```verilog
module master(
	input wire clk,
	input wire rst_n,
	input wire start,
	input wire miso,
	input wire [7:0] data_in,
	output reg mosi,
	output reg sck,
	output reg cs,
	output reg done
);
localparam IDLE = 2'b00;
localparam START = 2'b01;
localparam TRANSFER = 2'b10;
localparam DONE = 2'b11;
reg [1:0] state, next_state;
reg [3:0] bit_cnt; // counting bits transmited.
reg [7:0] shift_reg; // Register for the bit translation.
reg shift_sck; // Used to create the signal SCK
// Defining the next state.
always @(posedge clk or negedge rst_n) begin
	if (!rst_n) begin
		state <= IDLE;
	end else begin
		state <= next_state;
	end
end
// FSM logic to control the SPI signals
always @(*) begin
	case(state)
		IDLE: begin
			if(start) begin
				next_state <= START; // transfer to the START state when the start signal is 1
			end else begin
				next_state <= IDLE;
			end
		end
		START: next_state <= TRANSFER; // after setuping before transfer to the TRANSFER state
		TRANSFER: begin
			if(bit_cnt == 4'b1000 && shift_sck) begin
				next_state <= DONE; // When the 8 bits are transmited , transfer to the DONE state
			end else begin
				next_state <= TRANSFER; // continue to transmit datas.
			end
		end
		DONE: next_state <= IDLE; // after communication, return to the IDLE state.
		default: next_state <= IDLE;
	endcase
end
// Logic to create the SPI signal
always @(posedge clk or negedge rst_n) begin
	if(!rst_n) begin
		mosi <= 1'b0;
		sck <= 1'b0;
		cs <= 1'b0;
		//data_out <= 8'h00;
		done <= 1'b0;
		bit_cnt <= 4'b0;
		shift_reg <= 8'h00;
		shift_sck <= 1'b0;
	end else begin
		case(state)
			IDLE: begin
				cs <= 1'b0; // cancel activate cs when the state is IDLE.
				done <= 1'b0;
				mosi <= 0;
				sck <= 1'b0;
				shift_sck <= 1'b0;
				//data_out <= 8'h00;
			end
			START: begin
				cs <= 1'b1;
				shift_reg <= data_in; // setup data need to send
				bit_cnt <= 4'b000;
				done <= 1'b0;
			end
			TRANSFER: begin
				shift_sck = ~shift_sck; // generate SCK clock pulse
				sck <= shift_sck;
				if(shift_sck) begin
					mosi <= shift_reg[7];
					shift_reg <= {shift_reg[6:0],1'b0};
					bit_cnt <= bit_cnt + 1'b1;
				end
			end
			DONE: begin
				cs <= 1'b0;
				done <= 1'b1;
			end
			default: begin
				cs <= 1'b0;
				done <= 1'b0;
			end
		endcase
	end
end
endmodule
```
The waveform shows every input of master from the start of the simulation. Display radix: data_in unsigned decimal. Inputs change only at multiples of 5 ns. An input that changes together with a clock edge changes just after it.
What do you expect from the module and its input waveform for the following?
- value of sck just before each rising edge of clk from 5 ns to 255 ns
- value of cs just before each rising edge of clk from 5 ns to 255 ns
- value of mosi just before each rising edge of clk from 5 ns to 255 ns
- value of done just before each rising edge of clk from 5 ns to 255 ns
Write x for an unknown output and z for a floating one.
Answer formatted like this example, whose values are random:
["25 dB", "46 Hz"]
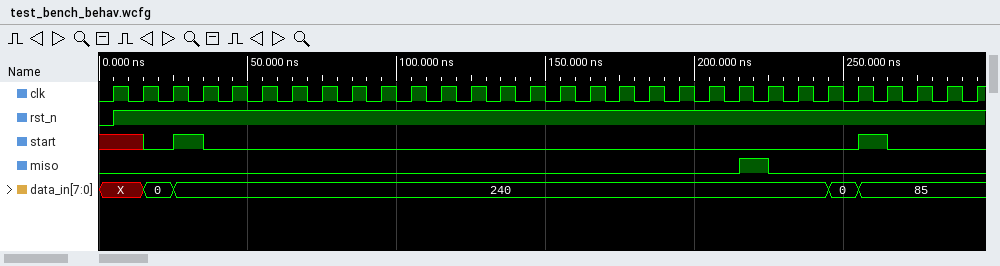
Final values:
["0 0 0 0 0 0 1 0 1 0 1 0 1 0 1 0 1 0 1 0 1 0 0 0 0 0", "0 0 0 0 0 1 1 1 1 1 1 1 1 1 1 1 1 1 1 1 1 1 0 0 0 0", "0 0 0 0 0 0 1 1 1 1 1 1 1 1 0 0 0 0 0 0 0 0 0 0 0 0", "0 0 0 0 0 0 0 0 0 0 0 0 0 0 0 0 0 0 0 0 0 0 1 0 0 0"]
